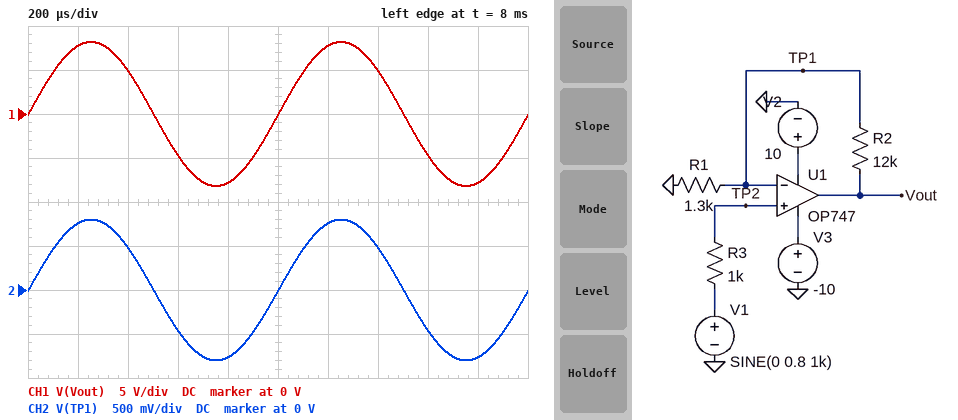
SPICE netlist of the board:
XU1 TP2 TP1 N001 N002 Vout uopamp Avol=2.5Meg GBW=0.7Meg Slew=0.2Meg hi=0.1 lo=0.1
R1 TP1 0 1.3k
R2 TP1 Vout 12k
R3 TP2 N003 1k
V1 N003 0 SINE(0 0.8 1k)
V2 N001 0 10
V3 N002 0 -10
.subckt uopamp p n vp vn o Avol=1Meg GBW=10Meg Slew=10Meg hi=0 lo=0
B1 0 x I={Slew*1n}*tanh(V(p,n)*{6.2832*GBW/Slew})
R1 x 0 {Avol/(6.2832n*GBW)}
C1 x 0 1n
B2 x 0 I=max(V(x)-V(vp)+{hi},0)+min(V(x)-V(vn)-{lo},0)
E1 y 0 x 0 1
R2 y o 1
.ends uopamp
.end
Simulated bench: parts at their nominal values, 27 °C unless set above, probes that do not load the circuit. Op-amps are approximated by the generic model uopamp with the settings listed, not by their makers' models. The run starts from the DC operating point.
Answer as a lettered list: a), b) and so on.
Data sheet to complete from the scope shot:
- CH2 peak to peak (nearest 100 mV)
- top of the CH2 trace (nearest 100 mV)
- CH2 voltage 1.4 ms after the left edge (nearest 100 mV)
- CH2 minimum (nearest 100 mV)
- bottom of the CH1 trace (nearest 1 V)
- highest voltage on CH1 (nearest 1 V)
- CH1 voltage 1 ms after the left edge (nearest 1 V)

a) 1.6 V
b) 800 mV
c) 500 mV
d) -800 mV
e) -8 V
f) 8 V
g) 0 V
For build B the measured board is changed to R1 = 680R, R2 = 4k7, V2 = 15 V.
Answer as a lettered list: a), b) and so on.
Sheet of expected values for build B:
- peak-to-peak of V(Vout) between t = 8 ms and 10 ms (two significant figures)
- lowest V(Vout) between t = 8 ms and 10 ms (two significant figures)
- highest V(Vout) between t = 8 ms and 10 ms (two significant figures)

a) 13 V
b) -6.3 V
c) 6.3 V
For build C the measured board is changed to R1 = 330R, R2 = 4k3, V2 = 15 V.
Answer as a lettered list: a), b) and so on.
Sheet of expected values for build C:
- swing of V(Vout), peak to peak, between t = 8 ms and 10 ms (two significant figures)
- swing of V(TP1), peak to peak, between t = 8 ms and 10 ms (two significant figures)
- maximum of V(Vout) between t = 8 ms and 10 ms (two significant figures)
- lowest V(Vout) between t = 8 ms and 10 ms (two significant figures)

a) 21 V
b) 1.5 V
c) 11 V
d) -9.9 V
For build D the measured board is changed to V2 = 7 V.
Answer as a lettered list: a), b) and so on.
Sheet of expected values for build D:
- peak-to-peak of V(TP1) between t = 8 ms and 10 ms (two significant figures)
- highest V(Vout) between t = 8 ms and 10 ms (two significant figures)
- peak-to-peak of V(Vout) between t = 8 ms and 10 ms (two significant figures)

a) 1.5 V
b) 6.9 V
c) 15 V
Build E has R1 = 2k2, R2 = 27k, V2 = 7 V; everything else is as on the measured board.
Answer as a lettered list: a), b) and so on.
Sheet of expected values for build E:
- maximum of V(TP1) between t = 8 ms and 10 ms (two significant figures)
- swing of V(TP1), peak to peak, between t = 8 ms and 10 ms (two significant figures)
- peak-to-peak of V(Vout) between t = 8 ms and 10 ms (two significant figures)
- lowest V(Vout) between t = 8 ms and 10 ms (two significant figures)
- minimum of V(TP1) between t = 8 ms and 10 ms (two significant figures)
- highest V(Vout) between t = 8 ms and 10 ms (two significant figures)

a) 520 mV
b) 1.3 V
c) 17 V
d) -9.9 V
e) -750 mV
f) 6.9 V
